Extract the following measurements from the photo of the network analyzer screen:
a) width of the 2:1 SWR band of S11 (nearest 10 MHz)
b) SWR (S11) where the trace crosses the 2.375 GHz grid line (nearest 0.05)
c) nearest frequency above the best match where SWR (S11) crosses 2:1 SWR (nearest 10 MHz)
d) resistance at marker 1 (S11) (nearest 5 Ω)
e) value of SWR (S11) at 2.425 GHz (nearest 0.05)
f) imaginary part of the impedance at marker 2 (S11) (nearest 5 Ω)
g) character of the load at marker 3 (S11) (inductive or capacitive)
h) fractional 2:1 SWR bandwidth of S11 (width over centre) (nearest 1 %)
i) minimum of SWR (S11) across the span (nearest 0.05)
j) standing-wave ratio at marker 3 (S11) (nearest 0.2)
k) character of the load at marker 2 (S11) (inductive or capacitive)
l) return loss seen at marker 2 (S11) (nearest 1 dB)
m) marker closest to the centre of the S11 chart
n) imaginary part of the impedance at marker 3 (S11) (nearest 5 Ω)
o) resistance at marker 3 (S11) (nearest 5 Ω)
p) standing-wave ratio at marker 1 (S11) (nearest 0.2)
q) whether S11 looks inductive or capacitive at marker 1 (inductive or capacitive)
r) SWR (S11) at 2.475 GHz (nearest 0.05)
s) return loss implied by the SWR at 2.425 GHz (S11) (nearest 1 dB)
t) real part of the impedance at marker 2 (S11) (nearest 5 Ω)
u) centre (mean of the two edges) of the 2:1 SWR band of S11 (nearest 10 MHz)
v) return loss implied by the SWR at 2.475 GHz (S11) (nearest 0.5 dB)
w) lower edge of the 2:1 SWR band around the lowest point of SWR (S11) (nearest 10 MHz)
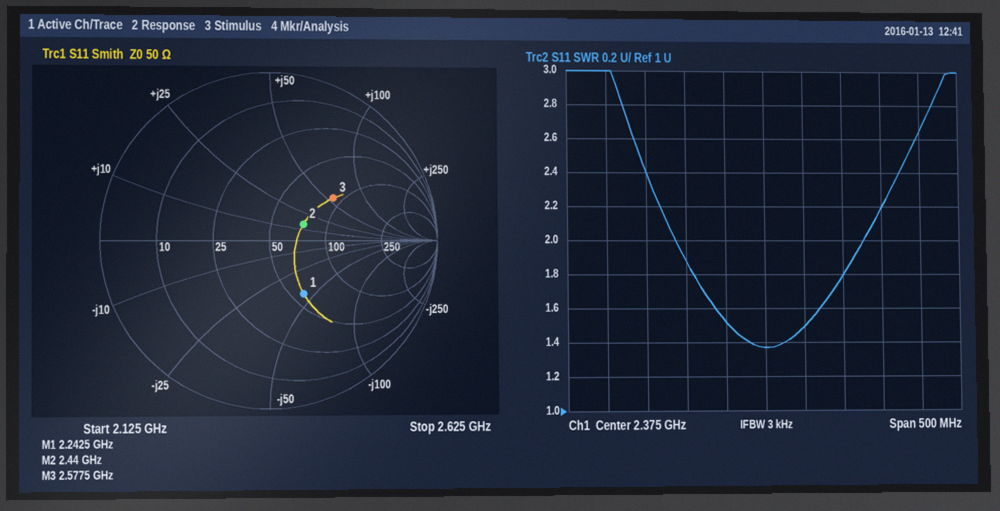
240 MHz
1.35
2.50 GHz
60 Ω
1.50
+15 Ω
inductive
10 %
1.35
2.6
inductive
13 dB
marker 2
+55 Ω
90 Ω
2.2
capacitive
1.80
14 dB
75 Ω
2.38 GHz
11.0 dB
2.26 GHz
